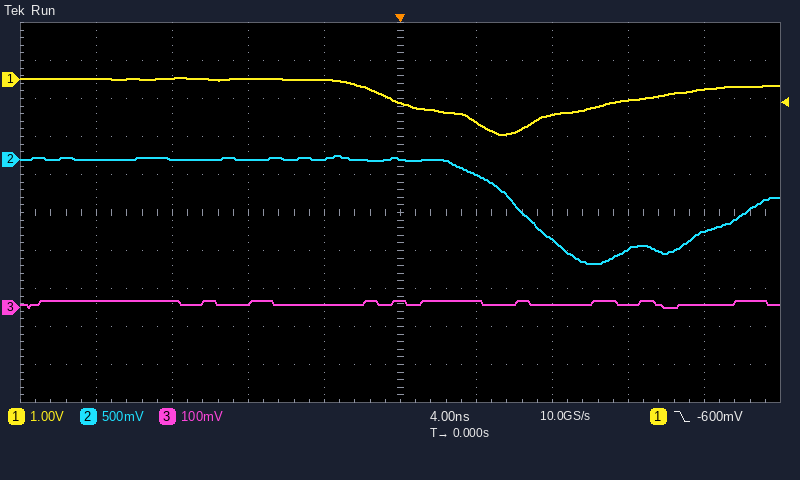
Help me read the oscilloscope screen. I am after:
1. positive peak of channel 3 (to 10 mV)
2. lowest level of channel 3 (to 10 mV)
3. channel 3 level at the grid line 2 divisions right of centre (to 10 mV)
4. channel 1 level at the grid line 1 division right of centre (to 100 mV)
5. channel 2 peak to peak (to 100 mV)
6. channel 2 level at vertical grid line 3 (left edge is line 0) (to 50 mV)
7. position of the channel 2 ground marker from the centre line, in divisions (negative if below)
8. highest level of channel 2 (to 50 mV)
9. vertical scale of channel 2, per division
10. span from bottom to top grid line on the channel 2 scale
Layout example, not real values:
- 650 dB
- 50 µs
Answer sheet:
- 20 mV
- 0 mV
- 10 mV
- -1.1 V
- 1.40 V
- 0 mV
- +1.4 div
- 50 mV
- 500 mV
- 5 V
